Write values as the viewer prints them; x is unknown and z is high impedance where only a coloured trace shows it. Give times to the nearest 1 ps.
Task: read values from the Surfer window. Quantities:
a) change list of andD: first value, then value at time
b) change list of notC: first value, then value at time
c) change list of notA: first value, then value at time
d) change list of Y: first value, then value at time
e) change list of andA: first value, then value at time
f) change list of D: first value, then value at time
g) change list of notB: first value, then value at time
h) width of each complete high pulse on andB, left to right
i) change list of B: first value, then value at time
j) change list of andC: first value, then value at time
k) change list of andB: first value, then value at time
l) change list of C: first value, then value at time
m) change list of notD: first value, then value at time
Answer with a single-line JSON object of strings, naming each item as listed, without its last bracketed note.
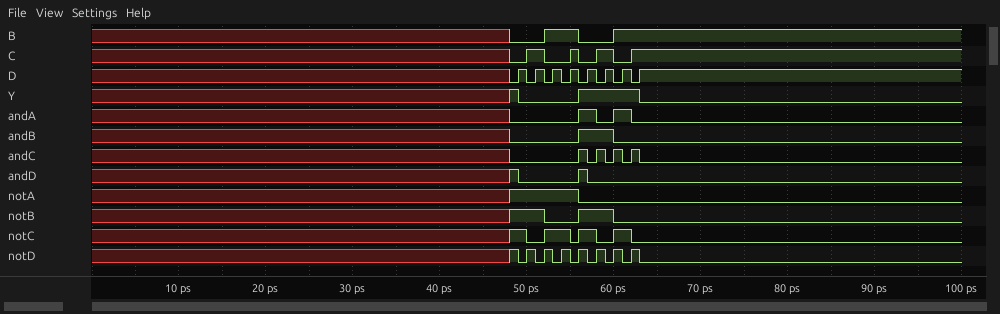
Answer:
{"change list of andD: first value, then value at time": "x, 1 at 48 ps, 0 at 49 ps, 1 at 56 ps, 0 at 57 ps", "change list of notC: first value, then value at time": "x, 1 at 48 ps, 0 at 50 ps, 1 at 52 ps, 0 at 55 ps, 1 at 56 ps, 0 at 58 ps, 1 at 60 ps, 0 at 62 ps", "change list of notA: first value, then value at time": "x, 1 at 48 ps, 0 at 56 ps", "change list of Y: first value, then value at time": "x, 1 at 48 ps, 0 at 49 ps, 1 at 56 ps, 0 at 63 ps", "change list of andA: first value, then value at time": "x, 0 at 48 ps, 1 at 56 ps, 0 at 58 ps, 1 at 60 ps, 0 at 62 ps", "change list of D: first value, then value at time": "x, 0 at 48 ps, 1 at 49 ps, 0 at 50 ps, 1 at 51 ps, 0 at 52 ps, 1 at 53 ps, 0 at 54 ps, 1 at 55 ps, 0 at 56 ps, 1 at 57 ps, 0 at 58 ps, 1 at 59 ps, 0 at 60 ps, 1 at 61 ps, 0 at 62 ps, 1 at 63 ps", "change list of notB: first value, then value at time": "x, 1 at 48 ps, 0 at 52 ps, 1 at 56 ps, 0 at 60 ps", "width of each complete high pulse on andB, left to right": "4 ps", "change list of B: first value, then value at time": "x, 0 at 48 ps, 1 at 52 ps, 0 at 56 ps, 1 at 60 ps", "change list of andC: first value, then value at time": "x, 0 at 48 ps, 1 at 56 ps, 0 at 57 ps, 1 at 58 ps, 0 at 59 ps, 1 at 60 ps, 0 at 61 ps, 1 at 62 ps, 0 at 63 ps", "change list of andB: first value, then value at time": "x, 0 at 48 ps, 1 at 56 ps, 0 at 60 ps", "change list of C: first value, then value at time": "x, 0 at 48 ps, 1 at 50 ps, 0 at 52 ps, 1 at 55 ps, 0 at 56 ps, 1 at 58 ps, 0 at 60 ps, 1 at 62 ps", "change list of notD: first value, then value at time": "x, 1 at 48 ps, 0 at 49 ps, 1 at 50 ps, 0 at 51 ps, 1 at 52 ps, 0 at 53 ps, 1 at 54 ps, 0 at 55 ps, 1 at 56 ps, 0 at 57 ps, 1 at 58 ps, 0 at 59 ps, 1 at 60 ps, 0 at 61 ps, 1 at 62 ps, 0 at 63 ps"}
